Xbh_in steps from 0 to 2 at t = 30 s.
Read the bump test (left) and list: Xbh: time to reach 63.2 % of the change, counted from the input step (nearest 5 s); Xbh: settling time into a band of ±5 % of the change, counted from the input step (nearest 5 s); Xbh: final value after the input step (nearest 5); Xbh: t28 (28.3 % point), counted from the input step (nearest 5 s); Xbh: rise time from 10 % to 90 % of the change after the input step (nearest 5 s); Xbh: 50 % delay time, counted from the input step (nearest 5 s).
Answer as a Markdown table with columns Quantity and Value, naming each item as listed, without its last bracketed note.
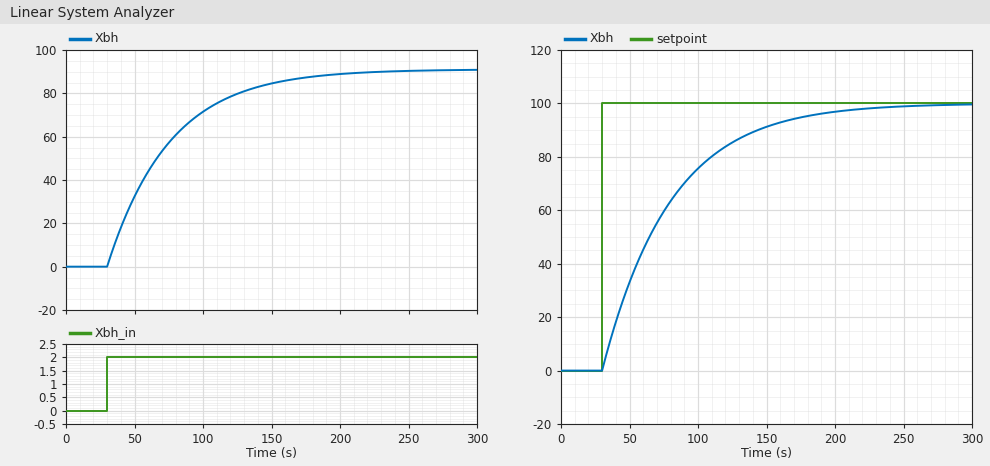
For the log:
| Quantity | Value |
|---|---|
| Xbh: time to reach 63.2 % of the change, counted from the input step | 45 s |
| Xbh: settling time into a band of ±5 % of the change, counted from the input step | 135 s |
| Xbh: final value after the input step | 90 |
| Xbh: t28 (28.3 % point), counted from the input step | 15 s |
| Xbh: rise time from 10 % to 90 % of the change after the input step | 100 s |
| Xbh: 50 % delay time, counted from the input step | 30 s |
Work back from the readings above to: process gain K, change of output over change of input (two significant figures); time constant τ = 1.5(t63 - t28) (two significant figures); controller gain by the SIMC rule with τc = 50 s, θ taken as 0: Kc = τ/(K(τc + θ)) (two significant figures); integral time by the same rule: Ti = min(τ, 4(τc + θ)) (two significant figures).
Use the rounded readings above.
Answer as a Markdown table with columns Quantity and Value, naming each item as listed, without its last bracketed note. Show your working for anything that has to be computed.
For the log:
| Quantity | Value |
|---|---|
| process gain K, change of output over change of input | (90 - 0) / 2 = 45 |
| time constant τ = 1.5(t63 - t28) | 1.5 × (45 - 15) = 45 s |
| controller gain by the SIMC rule with τc = 50 s, θ taken as 0: Kc = τ/(K(τc + θ)) | 45 / (45 × (50 + 0)) = 0.020 |
| integral time by the same rule: Ti = min(τ, 4(τc + θ)) | min(45, 4 × (50 + 0)) = 45 s |
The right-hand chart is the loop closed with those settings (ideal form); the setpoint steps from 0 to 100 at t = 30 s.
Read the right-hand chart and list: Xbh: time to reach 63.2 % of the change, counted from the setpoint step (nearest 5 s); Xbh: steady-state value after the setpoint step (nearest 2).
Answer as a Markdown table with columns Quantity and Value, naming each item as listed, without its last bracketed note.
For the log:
| Quantity | Value |
|---|---|
| Xbh: time to reach 63.2 % of the change, counted from the setpoint step | 50 s |
| Xbh: steady-state value after the setpoint step | 100 |
